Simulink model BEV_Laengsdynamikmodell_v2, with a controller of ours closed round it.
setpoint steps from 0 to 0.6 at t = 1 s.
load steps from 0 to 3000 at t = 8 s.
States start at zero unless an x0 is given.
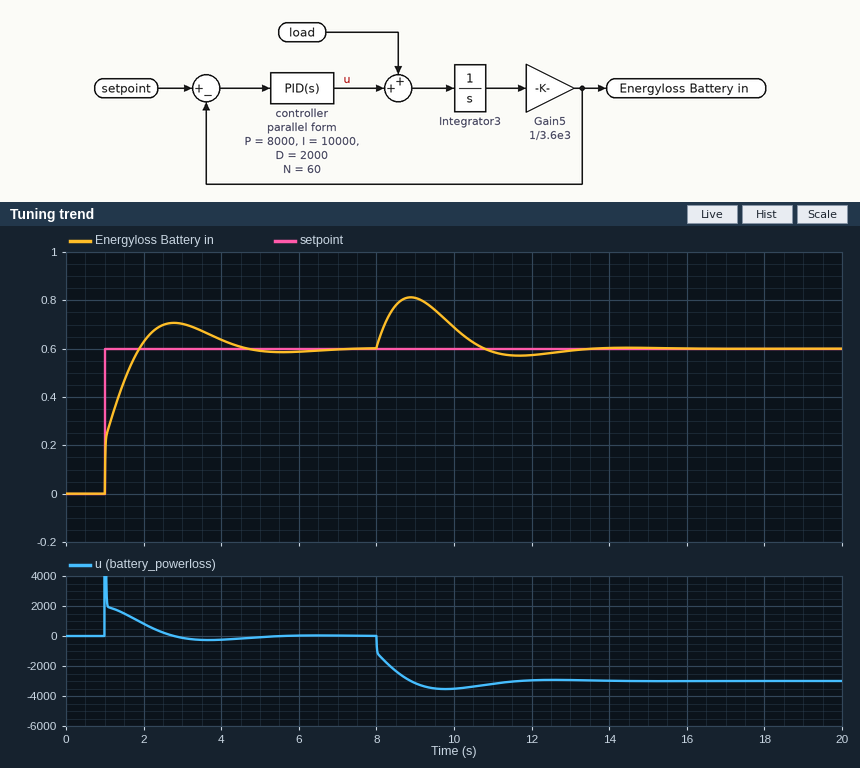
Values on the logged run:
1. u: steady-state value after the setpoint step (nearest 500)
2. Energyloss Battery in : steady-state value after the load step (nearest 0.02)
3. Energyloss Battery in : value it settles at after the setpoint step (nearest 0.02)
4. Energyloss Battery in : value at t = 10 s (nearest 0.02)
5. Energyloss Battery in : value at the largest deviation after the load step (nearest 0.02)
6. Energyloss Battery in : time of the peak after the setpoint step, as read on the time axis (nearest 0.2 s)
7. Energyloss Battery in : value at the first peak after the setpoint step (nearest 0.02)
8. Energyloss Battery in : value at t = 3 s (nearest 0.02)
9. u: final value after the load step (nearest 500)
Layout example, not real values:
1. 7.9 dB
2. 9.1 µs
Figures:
1. 0
2. 0.60
3. 0.60
4. 0.68
5. 0.82
6. 2.8 s
7. 0.70
8. 0.70
9. -3000
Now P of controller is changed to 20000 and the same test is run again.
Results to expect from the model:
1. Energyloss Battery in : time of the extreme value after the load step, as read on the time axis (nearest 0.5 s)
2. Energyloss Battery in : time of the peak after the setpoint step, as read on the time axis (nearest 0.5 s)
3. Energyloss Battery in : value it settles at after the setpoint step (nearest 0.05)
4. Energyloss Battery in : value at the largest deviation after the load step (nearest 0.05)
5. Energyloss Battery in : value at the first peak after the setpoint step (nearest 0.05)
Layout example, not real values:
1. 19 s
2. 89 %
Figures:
1. 8.5 s
2. 2.5 s
3. 0.60
4. 0.70
5. 0.65
